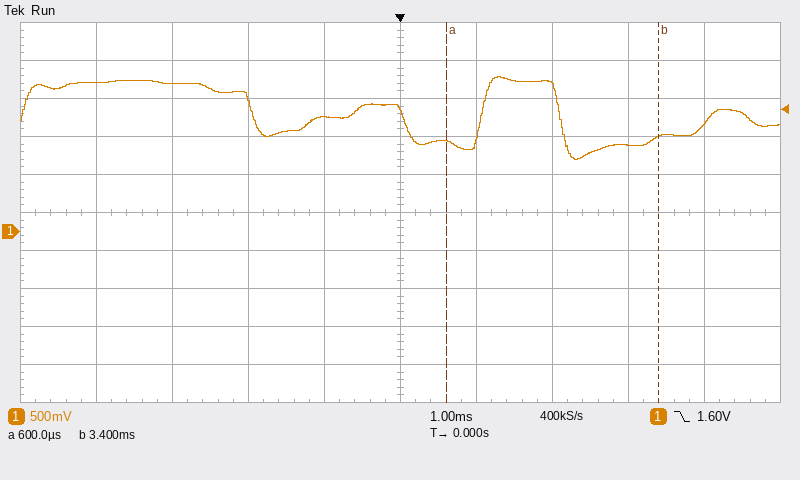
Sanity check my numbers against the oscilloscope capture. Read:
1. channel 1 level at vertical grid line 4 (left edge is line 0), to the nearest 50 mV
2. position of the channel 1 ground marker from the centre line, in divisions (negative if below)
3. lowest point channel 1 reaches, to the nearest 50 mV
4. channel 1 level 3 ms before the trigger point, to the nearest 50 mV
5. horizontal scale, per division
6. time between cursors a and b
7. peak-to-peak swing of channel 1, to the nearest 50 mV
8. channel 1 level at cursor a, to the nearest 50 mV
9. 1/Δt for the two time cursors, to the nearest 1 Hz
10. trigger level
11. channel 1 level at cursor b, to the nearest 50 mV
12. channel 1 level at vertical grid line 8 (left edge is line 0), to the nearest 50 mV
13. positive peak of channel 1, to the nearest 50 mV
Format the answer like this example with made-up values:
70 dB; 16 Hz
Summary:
1.50 V; -0.5 div; 950 mV; 1.95 V; 1 ms; 2.8 ms; 1.10 V; 1.20 V; 357 Hz; 1.60 V; 1.25 V; 1.15 V; 2.05 V
